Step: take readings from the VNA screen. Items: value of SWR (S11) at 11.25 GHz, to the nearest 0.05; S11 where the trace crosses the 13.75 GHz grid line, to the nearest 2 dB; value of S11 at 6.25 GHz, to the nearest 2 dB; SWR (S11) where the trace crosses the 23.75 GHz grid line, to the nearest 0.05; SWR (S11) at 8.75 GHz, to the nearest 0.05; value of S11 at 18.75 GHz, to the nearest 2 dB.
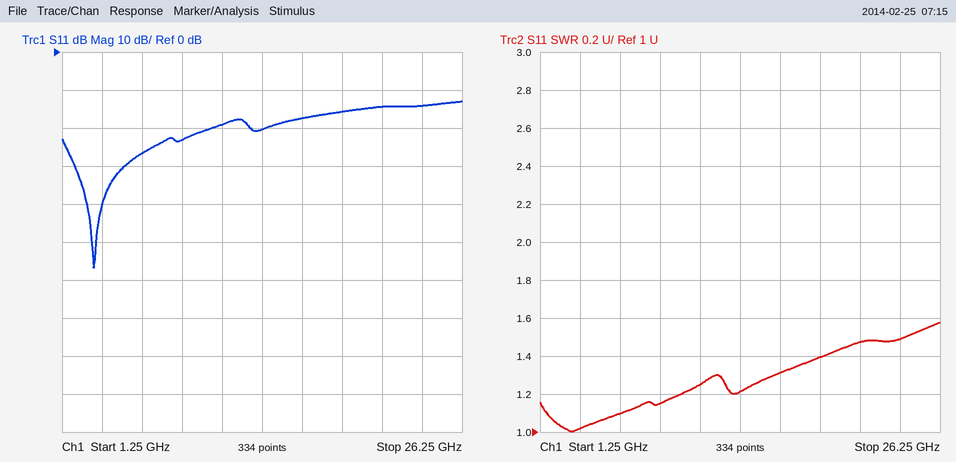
1.25
-20 dB
-26 dB
1.50
1.15
-16 dB
